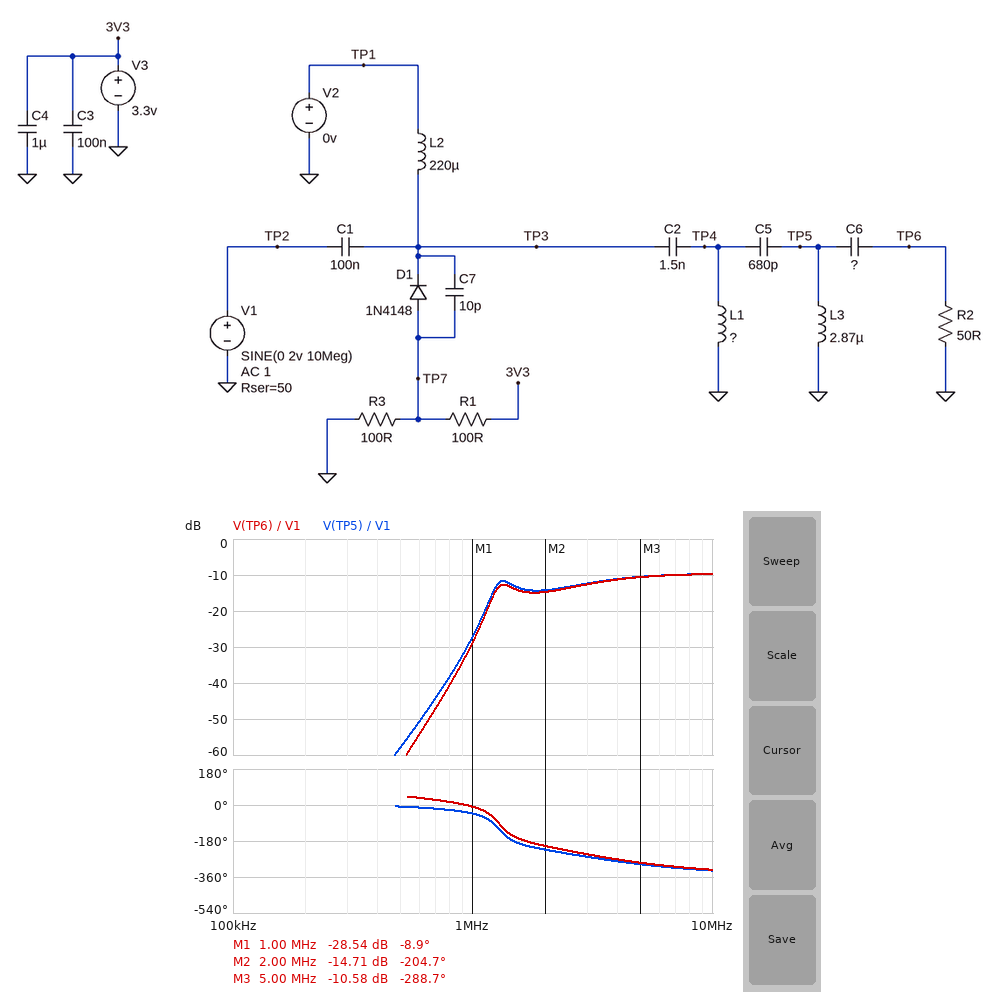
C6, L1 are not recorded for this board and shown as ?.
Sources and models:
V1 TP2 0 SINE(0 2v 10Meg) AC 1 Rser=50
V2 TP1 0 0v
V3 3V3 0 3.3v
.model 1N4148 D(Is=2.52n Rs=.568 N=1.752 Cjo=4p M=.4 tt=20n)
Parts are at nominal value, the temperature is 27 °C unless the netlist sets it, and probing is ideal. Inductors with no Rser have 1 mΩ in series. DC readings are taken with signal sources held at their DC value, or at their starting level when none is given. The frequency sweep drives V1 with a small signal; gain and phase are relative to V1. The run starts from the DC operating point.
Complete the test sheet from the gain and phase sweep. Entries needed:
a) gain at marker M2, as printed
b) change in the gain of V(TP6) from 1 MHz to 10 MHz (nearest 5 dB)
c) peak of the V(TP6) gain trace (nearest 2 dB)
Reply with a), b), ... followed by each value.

a) -14.71 dB
b) 20 dB
c) -10 dB
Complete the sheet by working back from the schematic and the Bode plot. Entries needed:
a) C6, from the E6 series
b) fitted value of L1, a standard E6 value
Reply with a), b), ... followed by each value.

a) 4.7 nF
b) 6.8 µH
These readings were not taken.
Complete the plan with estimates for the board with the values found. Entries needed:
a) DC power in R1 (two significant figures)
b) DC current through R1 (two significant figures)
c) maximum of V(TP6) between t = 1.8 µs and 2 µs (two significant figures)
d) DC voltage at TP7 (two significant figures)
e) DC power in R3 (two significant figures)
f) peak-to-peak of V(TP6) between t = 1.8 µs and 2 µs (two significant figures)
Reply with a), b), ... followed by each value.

a) 66 mW
b) 26 mA
c) 650 mV
d) 730 mV
e) 5.3 mW
f) 1.3 V
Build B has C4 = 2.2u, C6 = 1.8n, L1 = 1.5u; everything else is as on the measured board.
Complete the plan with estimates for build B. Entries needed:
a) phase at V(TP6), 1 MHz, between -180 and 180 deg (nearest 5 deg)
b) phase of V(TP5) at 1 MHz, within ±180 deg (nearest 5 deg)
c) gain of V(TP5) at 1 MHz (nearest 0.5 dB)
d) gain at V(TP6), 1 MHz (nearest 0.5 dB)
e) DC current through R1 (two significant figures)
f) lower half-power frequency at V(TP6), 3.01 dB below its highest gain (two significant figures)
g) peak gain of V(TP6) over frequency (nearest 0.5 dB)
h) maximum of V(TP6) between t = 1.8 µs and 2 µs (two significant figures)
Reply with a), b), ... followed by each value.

a) 40 deg
b) -20 deg
c) -46.0 dB
d) -52.0 dB
e) 26 mA
f) 2.3 MHz
g) -9.0 dB
h) 660 mV
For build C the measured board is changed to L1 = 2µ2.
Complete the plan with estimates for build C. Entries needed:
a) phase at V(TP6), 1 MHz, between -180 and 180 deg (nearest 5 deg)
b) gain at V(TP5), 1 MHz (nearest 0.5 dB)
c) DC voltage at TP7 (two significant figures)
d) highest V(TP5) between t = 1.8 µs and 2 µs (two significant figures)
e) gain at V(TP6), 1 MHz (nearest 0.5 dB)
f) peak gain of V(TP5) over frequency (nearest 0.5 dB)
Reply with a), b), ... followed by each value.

a) 0 deg
b) -42.0 dB
c) 730 mV
d) 670 mV
e) -44.0 dB
f) -9.0 dB
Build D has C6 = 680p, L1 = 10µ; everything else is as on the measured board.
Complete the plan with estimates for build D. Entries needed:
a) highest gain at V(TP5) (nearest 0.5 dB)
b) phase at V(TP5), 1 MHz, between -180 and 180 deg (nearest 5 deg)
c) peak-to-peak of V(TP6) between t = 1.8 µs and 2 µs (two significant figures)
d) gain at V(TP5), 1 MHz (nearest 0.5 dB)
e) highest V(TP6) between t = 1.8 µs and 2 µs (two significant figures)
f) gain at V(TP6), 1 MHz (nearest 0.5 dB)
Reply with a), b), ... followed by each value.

a) -4.5 dB
b) -55 deg
c) 1.2 V
d) -17.5 dB
e) 590 mV
f) -31.0 dB
